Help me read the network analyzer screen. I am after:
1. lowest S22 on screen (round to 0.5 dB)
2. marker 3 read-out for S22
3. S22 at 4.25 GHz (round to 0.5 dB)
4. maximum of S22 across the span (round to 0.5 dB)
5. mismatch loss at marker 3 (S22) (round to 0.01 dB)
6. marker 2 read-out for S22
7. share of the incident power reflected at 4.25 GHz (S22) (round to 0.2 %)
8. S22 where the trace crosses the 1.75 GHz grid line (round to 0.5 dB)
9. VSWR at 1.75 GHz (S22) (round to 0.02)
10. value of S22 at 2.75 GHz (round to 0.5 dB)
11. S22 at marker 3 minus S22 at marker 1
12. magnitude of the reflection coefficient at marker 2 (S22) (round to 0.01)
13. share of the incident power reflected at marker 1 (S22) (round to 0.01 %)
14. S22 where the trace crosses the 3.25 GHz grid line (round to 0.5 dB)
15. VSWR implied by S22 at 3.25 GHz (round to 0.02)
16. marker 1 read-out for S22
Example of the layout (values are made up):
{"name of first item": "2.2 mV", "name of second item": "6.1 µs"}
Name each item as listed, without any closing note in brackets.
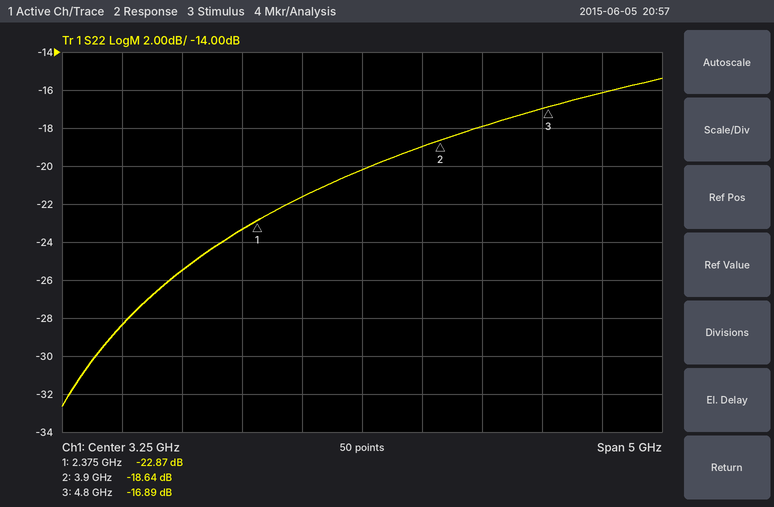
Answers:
{"lowest S22 on screen": "-32.5 dB", "marker 3 read-out for S22": "-16.89 dB", "S22 at 4.25 GHz": "-18.0 dB", "maximum of S22 across the span": "-15.5 dB", "mismatch loss at marker 3 (S22)": "0.09 dB", "marker 2 read-out for S22": "-18.64 dB", "share of the incident power reflected at 4.25 GHz (S22)": "1.6 %", "S22 where the trace crosses the 1.75 GHz grid line": "-25.5 dB", "VSWR at 1.75 GHz (S22)": "1.12", "value of S22 at 2.75 GHz": "-21.5 dB", "S22 at marker 3 minus S22 at marker 1": "5.98 dB", "magnitude of the reflection coefficient at marker 2 (S22)": "0.12", "share of the incident power reflected at marker 1 (S22)": "0.52 %", "S22 where the trace crosses the 3.25 GHz grid line": "-20.0 dB", "VSWR implied by S22 at 3.25 GHz": "1.22", "marker 1 read-out for S22": "-22.87 dB"}
